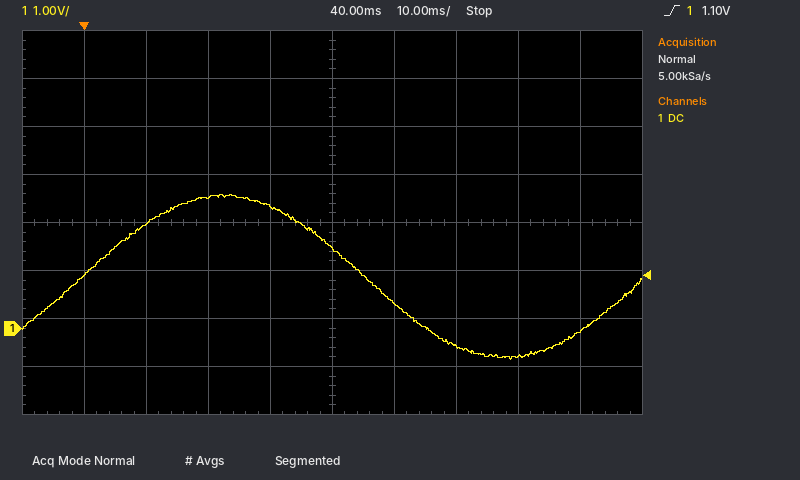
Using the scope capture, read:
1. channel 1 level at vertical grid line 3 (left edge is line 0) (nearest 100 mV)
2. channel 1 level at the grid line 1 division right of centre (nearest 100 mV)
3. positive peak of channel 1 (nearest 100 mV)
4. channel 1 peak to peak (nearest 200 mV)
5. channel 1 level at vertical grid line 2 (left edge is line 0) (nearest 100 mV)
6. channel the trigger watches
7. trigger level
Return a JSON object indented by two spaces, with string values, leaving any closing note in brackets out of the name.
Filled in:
{
  "channel 1 level at vertical grid line 3 (left edge is line 0)": "2.7 V",
  "channel 1 level at the grid line 1 division right of centre": "500 mV",
  "positive peak of channel 1": "2.8 V",
  "channel 1 peak to peak": "3.4 V",
  "channel 1 level at vertical grid line 2 (left edge is line 0)": "2.2 V",
  "channel the trigger watches": "channel 1",
  "trigger level": "1.10 V"
}
